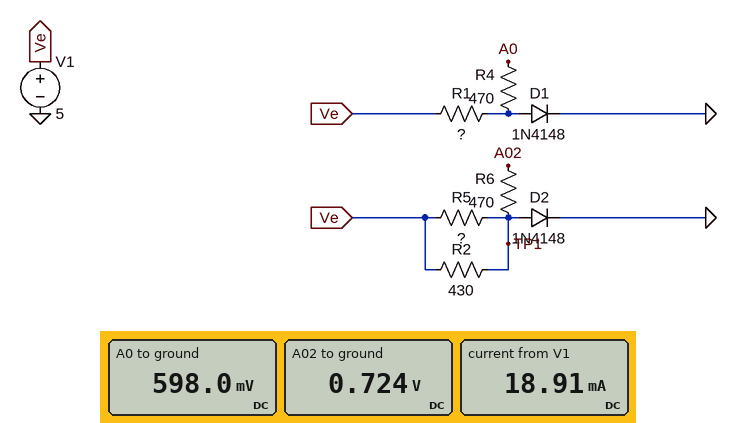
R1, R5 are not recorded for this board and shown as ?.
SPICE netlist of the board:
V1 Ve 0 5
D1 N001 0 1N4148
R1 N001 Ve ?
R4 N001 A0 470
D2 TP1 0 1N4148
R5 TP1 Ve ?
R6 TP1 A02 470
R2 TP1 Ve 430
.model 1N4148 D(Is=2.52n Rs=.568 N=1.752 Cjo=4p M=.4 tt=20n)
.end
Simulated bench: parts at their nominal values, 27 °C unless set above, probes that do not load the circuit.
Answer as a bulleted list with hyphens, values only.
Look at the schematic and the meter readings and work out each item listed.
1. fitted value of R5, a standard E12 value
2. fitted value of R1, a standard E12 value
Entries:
- 560 Ω
- 3.3 kΩ
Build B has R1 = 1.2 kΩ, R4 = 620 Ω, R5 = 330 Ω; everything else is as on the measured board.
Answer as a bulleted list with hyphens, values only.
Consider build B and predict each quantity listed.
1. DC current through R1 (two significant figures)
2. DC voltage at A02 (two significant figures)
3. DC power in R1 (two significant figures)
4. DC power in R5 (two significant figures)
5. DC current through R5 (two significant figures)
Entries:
- 3.6 mA
- 740 mV
- 16 mW
- 55 mW
- 13 mA
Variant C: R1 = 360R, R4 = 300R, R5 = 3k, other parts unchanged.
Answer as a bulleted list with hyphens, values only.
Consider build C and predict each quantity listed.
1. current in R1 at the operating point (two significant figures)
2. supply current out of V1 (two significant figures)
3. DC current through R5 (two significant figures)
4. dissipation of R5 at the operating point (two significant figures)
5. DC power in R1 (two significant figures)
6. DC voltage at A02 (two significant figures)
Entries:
- 12 mA
- 23 mA
- 1.4 mA
- 6.2 mW
- 51 mW
- 700 mV
